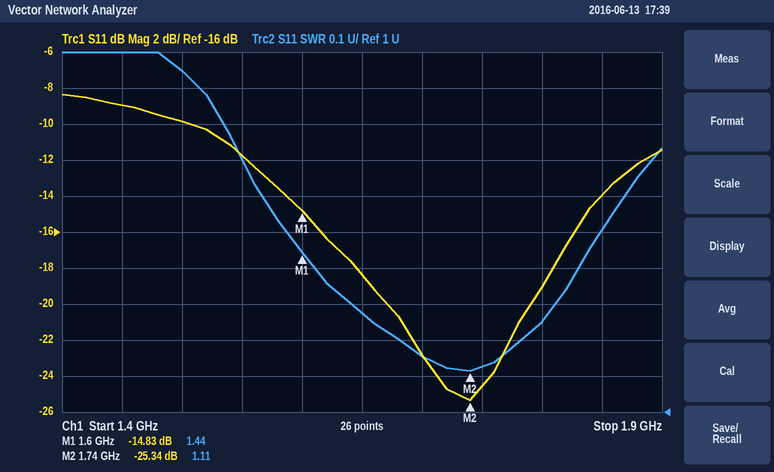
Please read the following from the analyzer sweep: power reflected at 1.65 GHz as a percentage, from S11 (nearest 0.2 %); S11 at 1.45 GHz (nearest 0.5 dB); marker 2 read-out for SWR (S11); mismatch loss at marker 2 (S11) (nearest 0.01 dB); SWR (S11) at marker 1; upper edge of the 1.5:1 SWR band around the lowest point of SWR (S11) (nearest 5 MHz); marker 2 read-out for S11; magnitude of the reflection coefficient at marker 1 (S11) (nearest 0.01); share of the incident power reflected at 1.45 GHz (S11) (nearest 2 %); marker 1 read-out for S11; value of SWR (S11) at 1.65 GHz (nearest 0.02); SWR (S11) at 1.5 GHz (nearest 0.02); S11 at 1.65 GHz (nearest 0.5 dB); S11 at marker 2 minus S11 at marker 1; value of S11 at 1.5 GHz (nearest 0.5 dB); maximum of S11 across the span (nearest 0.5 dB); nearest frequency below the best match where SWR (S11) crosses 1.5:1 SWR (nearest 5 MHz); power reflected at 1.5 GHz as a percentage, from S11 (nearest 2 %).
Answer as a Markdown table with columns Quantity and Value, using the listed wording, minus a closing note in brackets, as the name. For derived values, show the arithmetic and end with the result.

| Quantity | Value |
|---|---|
| power reflected at 1.65 GHz as a percentage, from S11 | 10^(-18.5/10) ≈ 1.4 % |
| S11 at 1.45 GHz | -9.0 dB |
| marker 2 read-out for SWR | 1.11 |
| mismatch loss at marker 2 (S11) | −10 log10(1 − 10^(-25.34/10)) ≈ 0.01 dB |
| SWR (S11) at marker 1 | 1.44 |
| upper edge of the 1.5:1 SWR band around the lowest point of SWR (S11) | 1.850 GHz |
| marker 2 read-out for S11 | -25.34 dB |
| magnitude of the reflection coefficient at marker 1 (S11) | 10^(-14.83/20) ≈ 0.18 |
| share of the incident power reflected at 1.45 GHz (S11) | 10^(-9/10) ≈ 12.6 %, so 12 % to the nearest 2 % |
| marker 1 read-out for S11 | -14.83 dB |
| value of SWR (S11) at 1.65 GHz | 1.28 |
| SWR (S11) at 1.5 GHz | 1.94 |
| S11 at 1.65 GHz | -18.5 dB |
| S11 at marker 2 minus S11 at marker 1 | -25.34 − (-14.83) = -10.51 dB |
| value of S11 at 1.5 GHz | -10.0 dB |
| maximum of S11 across the span | -8.5 dB |
| nearest frequency below the best match where SWR (S11) crosses 1.5:1 SWR | 1.585 GHz |
| power reflected at 1.5 GHz as a percentage, from S11 | 10^(-10/10) ≈ 10 % |
